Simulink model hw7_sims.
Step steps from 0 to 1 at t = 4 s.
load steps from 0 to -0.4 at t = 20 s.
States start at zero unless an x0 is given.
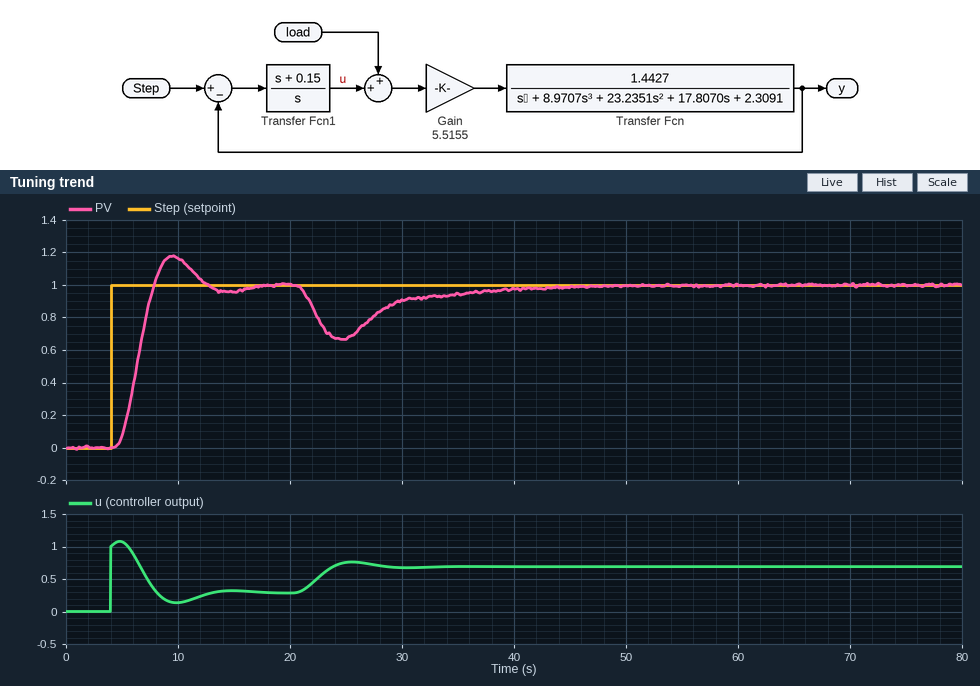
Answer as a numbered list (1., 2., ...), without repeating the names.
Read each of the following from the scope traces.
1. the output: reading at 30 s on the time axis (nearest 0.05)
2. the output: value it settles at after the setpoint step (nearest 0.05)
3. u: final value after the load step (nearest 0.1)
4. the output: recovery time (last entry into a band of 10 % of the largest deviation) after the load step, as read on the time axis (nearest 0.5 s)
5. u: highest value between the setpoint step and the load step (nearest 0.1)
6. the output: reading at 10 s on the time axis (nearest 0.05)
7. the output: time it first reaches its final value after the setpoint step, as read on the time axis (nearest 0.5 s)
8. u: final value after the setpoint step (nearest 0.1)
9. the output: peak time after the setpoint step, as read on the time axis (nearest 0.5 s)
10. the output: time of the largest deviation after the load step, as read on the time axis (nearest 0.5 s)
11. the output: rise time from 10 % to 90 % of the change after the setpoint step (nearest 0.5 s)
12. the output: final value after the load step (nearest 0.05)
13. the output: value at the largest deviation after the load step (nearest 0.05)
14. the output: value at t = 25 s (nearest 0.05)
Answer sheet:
1. 0.90
2. 1.00
3. 0.7
4. 38.5 s
5. 1.1
6. 1.15
7. 8.0 s
8. 0.3
9. 9.5 s
10. 24.5 s
11. 2.5 s
12. 1.00
13. 0.65
14. 0.65
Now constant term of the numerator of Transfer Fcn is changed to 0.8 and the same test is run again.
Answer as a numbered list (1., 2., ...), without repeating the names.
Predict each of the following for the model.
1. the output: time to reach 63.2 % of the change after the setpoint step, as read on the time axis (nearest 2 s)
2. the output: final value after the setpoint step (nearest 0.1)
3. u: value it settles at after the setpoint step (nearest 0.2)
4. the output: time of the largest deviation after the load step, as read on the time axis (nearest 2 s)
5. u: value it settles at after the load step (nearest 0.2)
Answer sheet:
1. 8 s
2. 1.0
3. 0.6
4. 26 s
5. 1.0
